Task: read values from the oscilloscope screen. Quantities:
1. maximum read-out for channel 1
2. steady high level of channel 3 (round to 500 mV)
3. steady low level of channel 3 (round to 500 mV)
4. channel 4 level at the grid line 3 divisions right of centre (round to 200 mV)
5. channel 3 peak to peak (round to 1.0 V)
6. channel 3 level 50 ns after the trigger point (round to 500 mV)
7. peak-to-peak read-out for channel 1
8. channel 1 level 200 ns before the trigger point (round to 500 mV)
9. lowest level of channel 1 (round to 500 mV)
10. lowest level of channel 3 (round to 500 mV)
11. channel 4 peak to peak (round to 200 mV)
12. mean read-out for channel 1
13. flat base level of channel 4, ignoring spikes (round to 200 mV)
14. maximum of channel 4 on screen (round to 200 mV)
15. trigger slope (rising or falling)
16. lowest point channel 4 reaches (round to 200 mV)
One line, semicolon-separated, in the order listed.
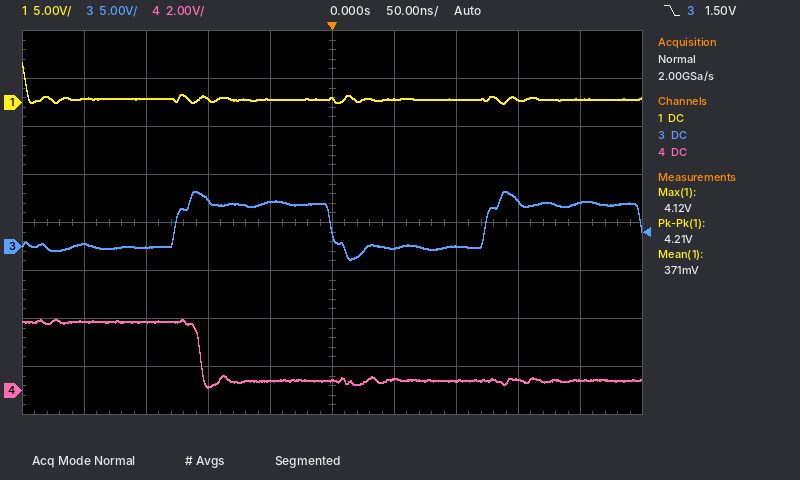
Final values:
4.12 V; 4.5 V; 0.0 V; 400 mV; 7.0 V; 0.0 V; 4.21 V; 500 mV; 0.0 V; -1.5 V; 2.8 V; 371 mV; 400 mV; 3.0 V; falling; 200 mV
